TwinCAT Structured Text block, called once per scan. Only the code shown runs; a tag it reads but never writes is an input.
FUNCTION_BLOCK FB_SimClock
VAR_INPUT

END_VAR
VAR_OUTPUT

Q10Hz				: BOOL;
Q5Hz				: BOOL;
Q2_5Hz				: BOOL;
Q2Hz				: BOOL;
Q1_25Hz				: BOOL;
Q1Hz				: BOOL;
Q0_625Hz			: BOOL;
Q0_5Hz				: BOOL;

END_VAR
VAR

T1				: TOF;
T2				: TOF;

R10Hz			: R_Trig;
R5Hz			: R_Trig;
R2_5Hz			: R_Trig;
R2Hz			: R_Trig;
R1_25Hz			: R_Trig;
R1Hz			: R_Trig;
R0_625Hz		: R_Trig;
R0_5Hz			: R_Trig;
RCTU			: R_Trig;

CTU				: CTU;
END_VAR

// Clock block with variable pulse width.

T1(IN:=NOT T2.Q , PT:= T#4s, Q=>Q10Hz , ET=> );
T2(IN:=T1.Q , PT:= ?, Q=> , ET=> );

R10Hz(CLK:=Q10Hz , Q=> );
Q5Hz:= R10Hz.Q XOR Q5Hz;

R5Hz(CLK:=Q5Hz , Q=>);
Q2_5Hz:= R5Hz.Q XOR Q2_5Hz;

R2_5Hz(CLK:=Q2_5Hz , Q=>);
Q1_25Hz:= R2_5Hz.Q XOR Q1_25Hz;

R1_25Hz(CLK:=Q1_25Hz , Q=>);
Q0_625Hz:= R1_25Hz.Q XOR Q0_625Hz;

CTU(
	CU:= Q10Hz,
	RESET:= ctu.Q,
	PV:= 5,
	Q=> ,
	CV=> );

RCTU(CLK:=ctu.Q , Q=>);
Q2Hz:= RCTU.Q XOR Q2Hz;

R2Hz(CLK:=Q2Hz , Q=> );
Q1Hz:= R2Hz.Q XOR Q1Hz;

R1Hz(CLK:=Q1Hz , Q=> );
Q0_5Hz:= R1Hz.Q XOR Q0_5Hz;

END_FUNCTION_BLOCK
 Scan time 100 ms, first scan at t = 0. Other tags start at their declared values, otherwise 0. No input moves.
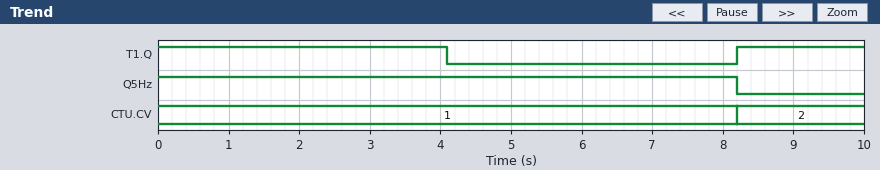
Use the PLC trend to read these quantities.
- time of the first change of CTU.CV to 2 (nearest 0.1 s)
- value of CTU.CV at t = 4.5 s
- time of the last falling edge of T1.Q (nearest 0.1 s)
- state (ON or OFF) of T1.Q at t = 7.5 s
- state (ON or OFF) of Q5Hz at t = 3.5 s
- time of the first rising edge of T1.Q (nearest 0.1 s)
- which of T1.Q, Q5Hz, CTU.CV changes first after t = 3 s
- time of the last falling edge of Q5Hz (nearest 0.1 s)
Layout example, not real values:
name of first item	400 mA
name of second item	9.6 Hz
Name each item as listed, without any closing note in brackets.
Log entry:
time of the first change of CTU.CV to 2	8.2 s
value of CTU.CV at t = 4.5 s	1
time of the last falling edge of T1.Q	4.1 s
state (ON or OFF) of T1.Q at t = 7.5 s	OFF
state (ON or OFF) of Q5Hz at t = 3.5 s	ON
time of the first rising edge of T1.Q	8.2 s
which of T1.Q, Q5Hz, CTU.CV changes first after t = 3 s	T1.Q
time of the last falling edge of Q5Hz	8.2 s
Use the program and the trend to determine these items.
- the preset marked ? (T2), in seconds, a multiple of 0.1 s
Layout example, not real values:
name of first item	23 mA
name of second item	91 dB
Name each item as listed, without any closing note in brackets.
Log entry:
the preset marked ? (T2), in seconds, a multiple of 0.1 s	4.0 s
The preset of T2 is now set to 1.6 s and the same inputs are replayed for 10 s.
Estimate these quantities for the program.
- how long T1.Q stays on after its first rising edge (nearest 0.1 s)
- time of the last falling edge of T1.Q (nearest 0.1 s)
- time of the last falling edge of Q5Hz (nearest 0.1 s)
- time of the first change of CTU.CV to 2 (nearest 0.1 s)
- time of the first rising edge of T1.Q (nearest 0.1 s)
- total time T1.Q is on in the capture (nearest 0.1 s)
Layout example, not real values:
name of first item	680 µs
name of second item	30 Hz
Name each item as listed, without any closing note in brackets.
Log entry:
how long T1.Q stays on after its first rising edge	4.1 s
time of the last falling edge of T1.Q	9.9 s
time of the last falling edge of Q5Hz	5.8 s
time of the first change of CTU.CV to 2	5.8 s
time of the first rising edge of T1.Q	5.8 s
total time T1.Q is on in the capture	8.2 s
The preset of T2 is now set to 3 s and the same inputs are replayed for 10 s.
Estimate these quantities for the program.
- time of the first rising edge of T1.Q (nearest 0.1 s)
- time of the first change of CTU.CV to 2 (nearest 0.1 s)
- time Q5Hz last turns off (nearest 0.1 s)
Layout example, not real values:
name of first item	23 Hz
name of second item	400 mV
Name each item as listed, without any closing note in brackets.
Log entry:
time of the first rising edge of T1.Q	7.2 s
time of the first change of CTU.CV to 2	7.2 s
time Q5Hz last turns off	7.2 s
